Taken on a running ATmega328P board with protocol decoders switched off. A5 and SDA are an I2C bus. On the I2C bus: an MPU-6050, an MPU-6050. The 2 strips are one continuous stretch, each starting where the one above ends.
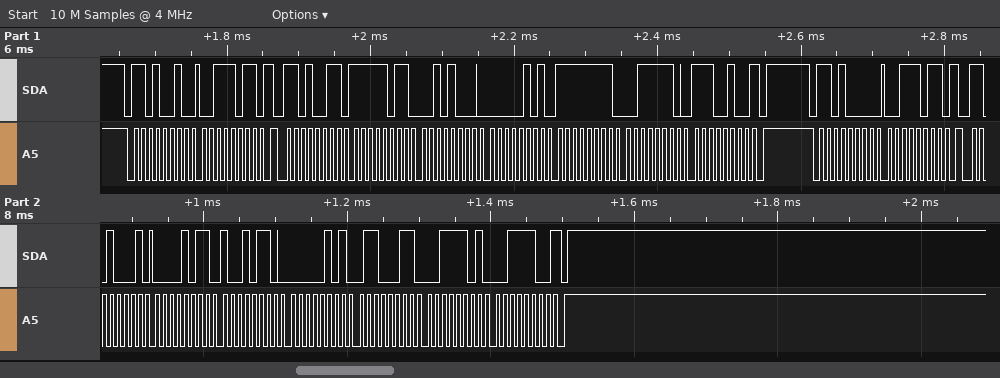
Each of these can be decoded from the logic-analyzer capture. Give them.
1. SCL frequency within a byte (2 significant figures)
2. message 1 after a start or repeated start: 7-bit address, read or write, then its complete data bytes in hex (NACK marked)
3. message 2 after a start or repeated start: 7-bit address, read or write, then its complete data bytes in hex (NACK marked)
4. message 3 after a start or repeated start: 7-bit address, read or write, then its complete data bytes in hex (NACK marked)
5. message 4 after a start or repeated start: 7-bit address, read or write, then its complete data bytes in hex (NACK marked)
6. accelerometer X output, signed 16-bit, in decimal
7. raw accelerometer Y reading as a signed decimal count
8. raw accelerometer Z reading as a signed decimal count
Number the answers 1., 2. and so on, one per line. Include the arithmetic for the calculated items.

1. 100 kHz
2. 0x69 write: 3B
3. 0x69 read: FB 28 05 FF 3E E4 NACK
4. 0x68 write: 3B
5. 0x68 read: 0B 96 05 63 3D 3C NACK
6. 0xFB28 = -1240
7. 0x05FF = 1535
8. 0x3EE4 = 16100
